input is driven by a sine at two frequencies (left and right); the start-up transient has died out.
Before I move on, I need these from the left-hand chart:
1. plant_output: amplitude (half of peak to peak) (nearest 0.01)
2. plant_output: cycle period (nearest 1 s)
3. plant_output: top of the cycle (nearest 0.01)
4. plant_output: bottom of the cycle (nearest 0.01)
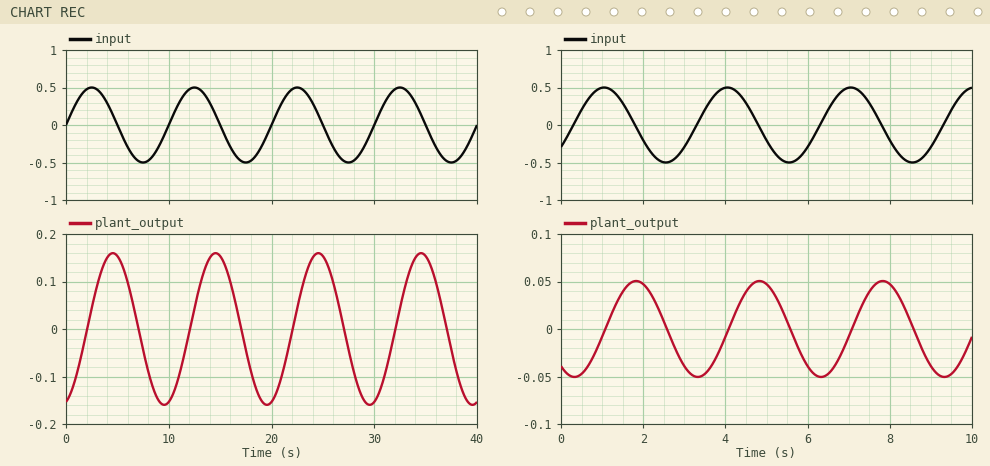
0.16
10 s
0.16
-0.16
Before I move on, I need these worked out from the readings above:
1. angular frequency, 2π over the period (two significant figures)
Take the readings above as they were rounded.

0.63 rad/s
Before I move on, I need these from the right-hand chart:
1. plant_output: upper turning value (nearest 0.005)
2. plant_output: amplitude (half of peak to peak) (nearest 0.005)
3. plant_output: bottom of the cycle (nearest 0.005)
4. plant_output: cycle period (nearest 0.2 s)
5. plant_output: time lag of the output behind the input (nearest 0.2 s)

0.050
0.050
-0.050
3.0 s
0.8 s
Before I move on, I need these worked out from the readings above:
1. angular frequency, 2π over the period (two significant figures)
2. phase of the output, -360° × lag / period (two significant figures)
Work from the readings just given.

2.1 rad/s
-96°
